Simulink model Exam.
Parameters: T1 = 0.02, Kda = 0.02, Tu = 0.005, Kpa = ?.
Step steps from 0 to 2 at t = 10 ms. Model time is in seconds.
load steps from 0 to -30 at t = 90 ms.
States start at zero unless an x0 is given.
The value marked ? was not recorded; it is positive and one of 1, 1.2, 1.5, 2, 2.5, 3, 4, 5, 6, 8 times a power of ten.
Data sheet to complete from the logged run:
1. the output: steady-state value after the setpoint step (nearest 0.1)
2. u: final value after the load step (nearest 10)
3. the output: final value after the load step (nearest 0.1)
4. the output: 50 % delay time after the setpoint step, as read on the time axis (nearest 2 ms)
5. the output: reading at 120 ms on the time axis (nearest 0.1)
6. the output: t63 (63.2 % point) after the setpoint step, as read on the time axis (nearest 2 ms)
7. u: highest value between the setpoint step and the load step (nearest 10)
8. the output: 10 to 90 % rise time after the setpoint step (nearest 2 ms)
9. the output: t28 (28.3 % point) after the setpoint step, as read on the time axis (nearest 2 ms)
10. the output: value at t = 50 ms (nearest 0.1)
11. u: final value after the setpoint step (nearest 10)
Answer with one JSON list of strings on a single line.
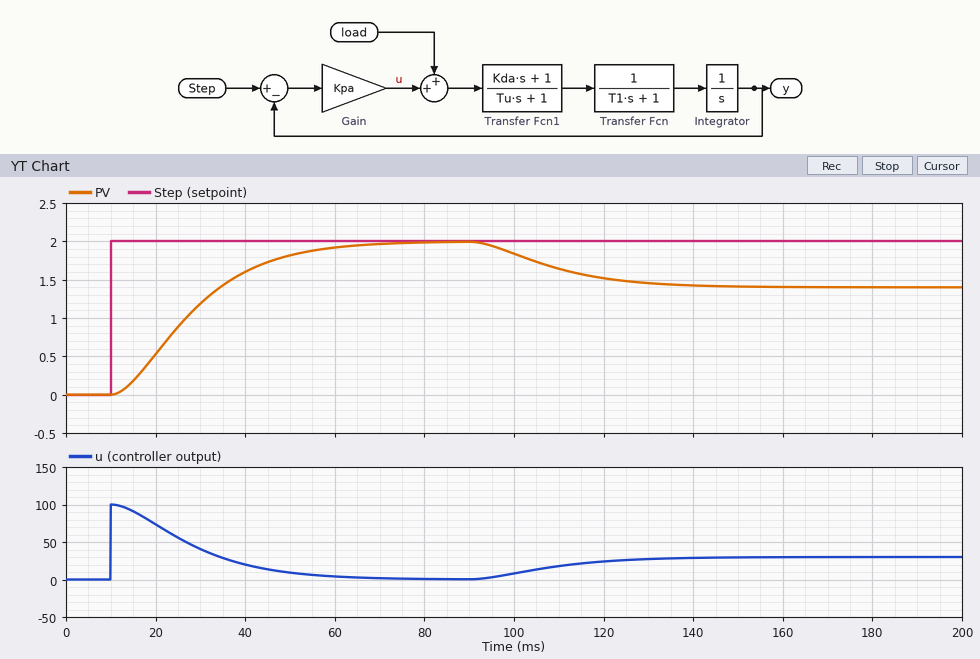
["2.0", "30", "1.4", "26 ms", "1.5", "32 ms", "100", "34 ms", "20 ms", "1.8", "0"]
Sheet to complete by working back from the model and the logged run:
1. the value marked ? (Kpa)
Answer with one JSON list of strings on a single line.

["50"]
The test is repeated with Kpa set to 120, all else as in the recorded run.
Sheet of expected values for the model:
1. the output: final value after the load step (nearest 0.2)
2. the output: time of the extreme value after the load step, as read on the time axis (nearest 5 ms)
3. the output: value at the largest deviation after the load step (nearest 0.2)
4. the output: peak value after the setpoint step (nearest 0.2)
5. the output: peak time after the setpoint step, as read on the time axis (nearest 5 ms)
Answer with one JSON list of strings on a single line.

["1.8", "115 ms", "1.8", "2.2", "35 ms"]
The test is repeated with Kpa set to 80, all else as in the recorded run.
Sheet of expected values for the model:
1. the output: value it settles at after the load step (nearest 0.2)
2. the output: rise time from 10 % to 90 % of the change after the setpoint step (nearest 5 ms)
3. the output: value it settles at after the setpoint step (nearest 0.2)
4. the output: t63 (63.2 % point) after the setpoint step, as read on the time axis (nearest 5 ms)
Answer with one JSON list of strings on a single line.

["1.6", "20 ms", "2.0", "25 ms"]
